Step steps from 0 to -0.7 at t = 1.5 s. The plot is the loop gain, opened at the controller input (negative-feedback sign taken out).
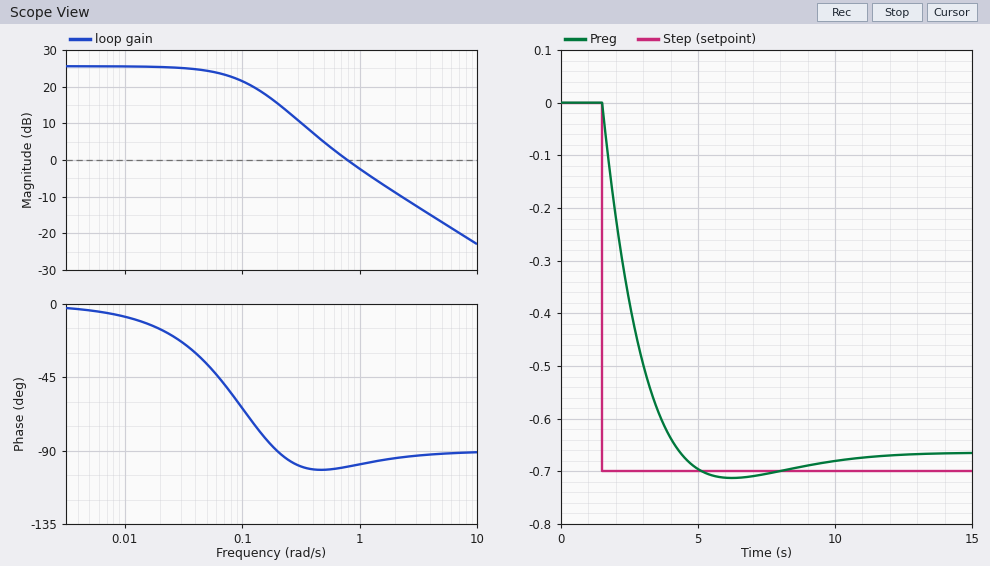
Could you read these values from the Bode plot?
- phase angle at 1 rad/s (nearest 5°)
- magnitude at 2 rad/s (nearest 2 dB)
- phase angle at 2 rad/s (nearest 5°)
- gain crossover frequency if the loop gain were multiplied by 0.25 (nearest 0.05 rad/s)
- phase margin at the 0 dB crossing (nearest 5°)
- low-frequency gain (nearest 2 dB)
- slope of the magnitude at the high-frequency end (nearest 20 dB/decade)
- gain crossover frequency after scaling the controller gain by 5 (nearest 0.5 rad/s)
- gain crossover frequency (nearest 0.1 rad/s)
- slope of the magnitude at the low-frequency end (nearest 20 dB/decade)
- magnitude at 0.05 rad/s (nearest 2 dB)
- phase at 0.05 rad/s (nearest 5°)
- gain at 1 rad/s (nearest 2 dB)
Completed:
-100°
-8 dB
-95°
0.25 rad/s
80°
26 dB
-20 dB/decade
3.5 rad/s
0.8 rad/s
0 dB/decade
24 dB
-35°
-2 dB
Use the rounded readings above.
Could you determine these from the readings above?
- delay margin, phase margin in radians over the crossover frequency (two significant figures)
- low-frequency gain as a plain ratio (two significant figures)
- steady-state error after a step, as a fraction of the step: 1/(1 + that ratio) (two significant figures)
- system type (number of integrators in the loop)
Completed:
1.7 s
20
0.048
0
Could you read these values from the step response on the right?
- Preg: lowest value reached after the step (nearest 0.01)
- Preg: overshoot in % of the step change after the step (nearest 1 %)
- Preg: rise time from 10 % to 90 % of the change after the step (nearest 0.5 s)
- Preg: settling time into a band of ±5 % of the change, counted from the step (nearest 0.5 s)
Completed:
-0.71
7 %
2.0 s
6.5 s
